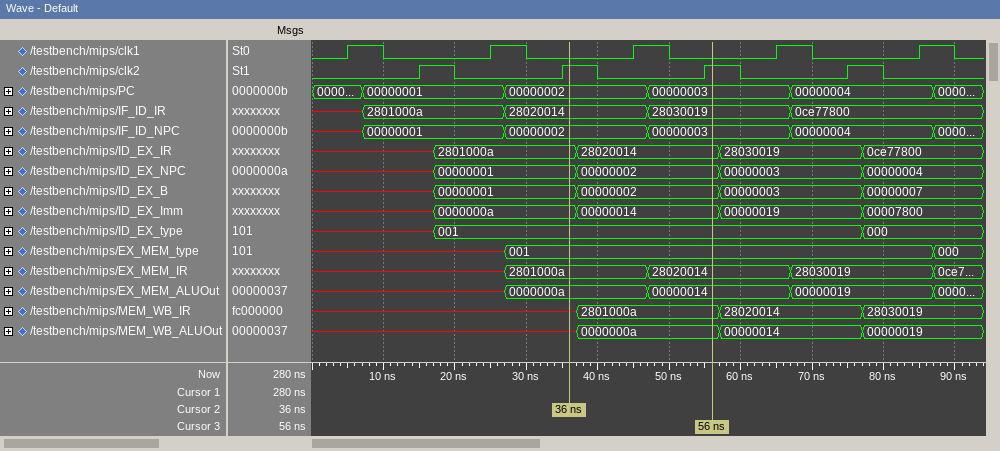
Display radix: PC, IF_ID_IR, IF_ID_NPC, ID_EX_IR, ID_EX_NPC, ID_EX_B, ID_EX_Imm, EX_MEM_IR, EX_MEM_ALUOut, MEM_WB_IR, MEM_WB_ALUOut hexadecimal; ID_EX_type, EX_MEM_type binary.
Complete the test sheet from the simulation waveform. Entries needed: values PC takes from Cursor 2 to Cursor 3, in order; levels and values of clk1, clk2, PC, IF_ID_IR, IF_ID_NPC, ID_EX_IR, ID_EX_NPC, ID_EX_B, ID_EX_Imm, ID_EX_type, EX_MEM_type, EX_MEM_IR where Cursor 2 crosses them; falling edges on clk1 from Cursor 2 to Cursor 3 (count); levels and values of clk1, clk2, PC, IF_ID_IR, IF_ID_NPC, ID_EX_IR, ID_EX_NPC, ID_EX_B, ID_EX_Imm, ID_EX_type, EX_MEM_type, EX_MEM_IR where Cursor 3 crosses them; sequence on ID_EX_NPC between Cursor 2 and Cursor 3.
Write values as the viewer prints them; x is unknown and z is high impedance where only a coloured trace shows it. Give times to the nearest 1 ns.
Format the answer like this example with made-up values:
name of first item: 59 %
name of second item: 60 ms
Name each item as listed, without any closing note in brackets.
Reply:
values PC takes from Cursor 2 to Cursor 3, in order: 00000002, 00000003
levels and values of clk1, clk2, PC, IF_ID_IR, IF_ID_NPC, ID_EX_IR, ID_EX_NPC, ID_EX_B, ID_EX_Imm, ID_EX_type, EX_MEM_type, EX_MEM_IR where Cursor 2 crosses them: clk1=0, clk2=1, PC=00000002, IF_ID_IR=28020014, IF_ID_NPC=00000002, ID_EX_IR=2801000a, ID_EX_NPC=00000001, ID_EX_B=00000001, ID_EX_Imm=0000000a, ID_EX_type=001, EX_MEM_type=001, EX_MEM_IR=2801000a
falling edges on clk1 from Cursor 2 to Cursor 3: 1
levels and values of clk1, clk2, PC, IF_ID_IR, IF_ID_NPC, ID_EX_IR, ID_EX_NPC, ID_EX_B, ID_EX_Imm, ID_EX_type, EX_MEM_type, EX_MEM_IR where Cursor 3 crosses them: clk1=0, clk2=1, PC=00000003, IF_ID_IR=28030019, IF_ID_NPC=00000003, ID_EX_IR=28020014, ID_EX_NPC=00000002, ID_EX_B=00000002, ID_EX_Imm=00000014, ID_EX_type=001, EX_MEM_type=001, EX_MEM_IR=28020014
sequence on ID_EX_NPC between Cursor 2 and Cursor 3: 00000001, 00000002
